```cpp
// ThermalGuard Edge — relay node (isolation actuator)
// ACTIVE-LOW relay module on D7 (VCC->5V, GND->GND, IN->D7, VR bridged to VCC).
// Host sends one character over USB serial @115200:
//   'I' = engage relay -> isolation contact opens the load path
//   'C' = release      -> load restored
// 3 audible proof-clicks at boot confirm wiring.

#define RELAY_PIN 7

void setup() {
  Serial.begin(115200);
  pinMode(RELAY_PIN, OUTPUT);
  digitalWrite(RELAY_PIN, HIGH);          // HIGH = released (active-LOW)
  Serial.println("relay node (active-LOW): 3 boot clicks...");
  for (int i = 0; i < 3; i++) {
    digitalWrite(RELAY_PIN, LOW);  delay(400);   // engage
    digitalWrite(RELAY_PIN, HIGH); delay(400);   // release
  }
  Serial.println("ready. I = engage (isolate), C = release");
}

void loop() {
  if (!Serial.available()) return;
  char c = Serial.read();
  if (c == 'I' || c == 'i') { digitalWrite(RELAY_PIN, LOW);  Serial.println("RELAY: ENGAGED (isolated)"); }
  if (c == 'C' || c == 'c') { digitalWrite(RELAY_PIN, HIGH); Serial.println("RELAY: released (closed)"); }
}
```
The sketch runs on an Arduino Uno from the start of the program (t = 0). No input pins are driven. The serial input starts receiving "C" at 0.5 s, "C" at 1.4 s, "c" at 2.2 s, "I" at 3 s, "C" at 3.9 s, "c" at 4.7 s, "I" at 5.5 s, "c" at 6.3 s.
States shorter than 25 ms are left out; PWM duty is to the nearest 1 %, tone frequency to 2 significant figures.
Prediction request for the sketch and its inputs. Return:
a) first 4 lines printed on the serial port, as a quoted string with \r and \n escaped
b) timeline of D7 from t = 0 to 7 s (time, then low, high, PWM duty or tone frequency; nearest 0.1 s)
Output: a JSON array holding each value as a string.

["\"relay node (active-LOW): 3 boot clicks...\\r\\nready. I = engage (isolate), C = release\\r\\nRELAY: released (closed)\\r\\nRELAY: released (closed)\\r\\n\"", "0 s low; 0.4 s high; 0.8 s low; 1.2 s high; 1.6 s low; 2 s high; 3 s low; 3.9 s high; 5.5 s low; 6.3 s high"]
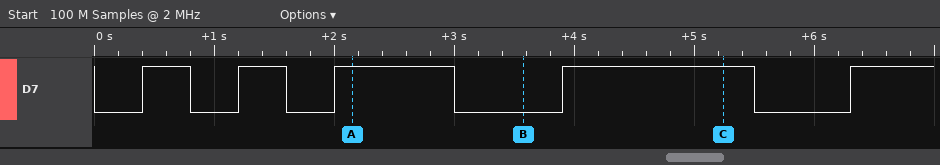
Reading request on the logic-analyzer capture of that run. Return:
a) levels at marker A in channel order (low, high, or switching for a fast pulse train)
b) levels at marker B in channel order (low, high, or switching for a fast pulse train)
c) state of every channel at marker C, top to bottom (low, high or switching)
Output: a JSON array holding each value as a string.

["D7 high", "D7 low", "D7 high"]
